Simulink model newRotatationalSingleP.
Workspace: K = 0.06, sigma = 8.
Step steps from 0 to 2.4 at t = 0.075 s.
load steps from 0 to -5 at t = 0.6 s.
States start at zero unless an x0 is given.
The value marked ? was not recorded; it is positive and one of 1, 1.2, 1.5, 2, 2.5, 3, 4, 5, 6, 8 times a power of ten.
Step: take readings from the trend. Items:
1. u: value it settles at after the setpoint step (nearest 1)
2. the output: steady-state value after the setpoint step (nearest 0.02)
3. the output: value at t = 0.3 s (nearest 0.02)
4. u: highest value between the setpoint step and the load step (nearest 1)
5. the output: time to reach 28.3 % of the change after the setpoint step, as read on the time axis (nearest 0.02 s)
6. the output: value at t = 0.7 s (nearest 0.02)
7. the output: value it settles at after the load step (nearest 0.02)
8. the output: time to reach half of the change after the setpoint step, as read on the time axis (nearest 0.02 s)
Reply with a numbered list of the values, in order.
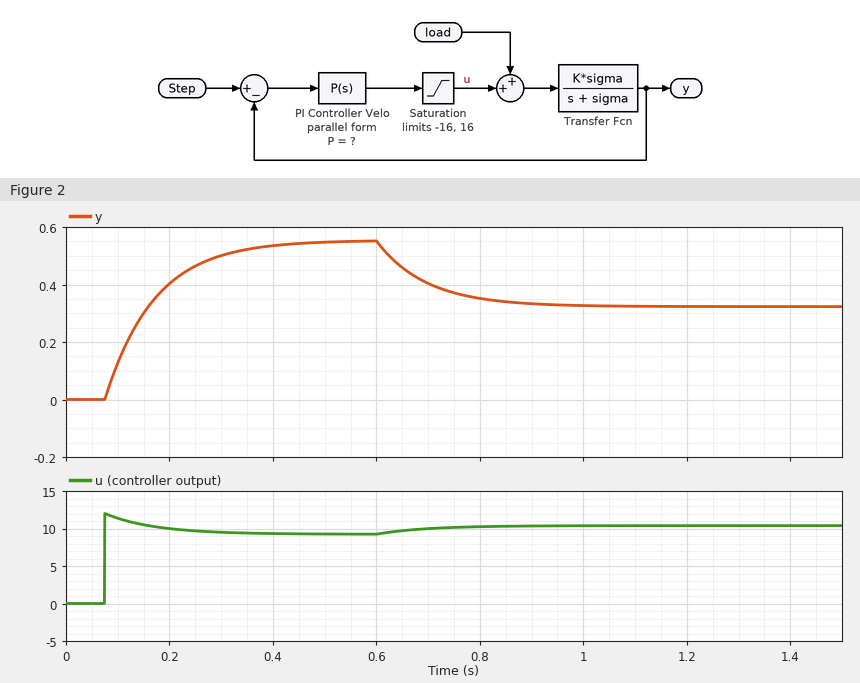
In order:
1. 9
2. 0.56
3. 0.50
4. 12
5. 0.10 s
6. 0.40
7. 0.32
8. 0.14 s
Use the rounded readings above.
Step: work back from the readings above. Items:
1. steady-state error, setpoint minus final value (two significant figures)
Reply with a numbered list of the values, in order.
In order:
1. 1.8
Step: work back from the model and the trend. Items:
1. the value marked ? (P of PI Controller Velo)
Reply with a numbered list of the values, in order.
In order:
1. 5
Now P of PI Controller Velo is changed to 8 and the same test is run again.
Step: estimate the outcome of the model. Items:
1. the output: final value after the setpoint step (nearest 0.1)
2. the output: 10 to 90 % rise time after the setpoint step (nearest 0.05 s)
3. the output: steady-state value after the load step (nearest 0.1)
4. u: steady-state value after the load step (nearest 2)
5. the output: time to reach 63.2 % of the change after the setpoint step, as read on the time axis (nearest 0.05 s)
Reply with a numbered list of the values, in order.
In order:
1. 0.8
2. 0.20 s
3. 0.6
4. 14
5. 0.15 s
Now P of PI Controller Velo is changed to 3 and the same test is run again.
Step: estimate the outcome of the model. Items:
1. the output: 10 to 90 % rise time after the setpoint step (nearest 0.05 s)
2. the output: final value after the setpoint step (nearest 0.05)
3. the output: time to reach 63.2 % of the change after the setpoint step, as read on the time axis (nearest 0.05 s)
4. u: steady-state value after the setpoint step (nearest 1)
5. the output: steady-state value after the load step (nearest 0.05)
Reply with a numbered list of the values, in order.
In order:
1. 0.25 s
2. 0.35
3. 0.20 s
4. 6
5. 0.10
